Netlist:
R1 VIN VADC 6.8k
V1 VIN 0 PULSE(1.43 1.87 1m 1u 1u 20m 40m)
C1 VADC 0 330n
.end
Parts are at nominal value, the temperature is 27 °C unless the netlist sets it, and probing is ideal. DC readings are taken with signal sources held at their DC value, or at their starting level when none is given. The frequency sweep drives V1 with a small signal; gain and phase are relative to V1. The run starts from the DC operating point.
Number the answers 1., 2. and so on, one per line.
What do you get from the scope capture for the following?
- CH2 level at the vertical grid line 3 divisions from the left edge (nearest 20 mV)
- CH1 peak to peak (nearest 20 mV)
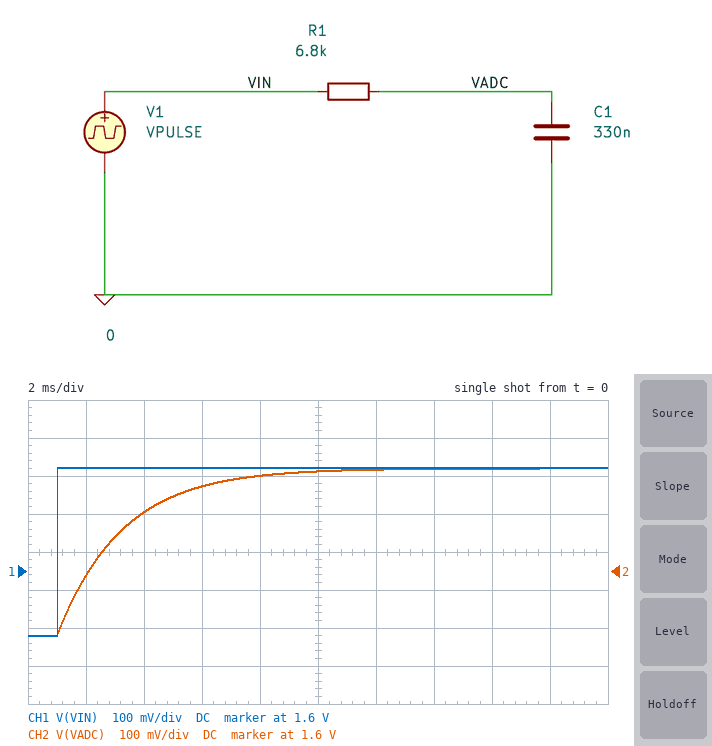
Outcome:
1. 1.82 V
2. 440 mV
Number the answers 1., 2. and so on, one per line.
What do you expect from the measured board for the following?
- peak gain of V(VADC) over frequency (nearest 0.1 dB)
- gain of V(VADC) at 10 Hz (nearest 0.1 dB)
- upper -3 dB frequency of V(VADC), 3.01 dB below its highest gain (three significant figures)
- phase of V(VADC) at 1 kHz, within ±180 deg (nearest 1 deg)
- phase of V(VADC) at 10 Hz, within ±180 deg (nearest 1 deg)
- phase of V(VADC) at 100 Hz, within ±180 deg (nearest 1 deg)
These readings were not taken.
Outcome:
1. 0 dB
2. -0.1 dB
3. 70.9 Hz
4. -86 deg
5. -8 deg
6. -55 deg
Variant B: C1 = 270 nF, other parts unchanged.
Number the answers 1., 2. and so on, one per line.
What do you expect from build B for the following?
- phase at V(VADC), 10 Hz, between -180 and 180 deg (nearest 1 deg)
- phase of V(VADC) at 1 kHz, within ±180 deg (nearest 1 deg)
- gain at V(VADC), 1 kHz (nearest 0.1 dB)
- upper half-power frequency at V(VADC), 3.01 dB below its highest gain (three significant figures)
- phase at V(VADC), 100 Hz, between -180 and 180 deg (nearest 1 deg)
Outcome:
1. -7 deg
2. -85 deg
3. -21.3 dB
4. 86.7 Hz
5. -49 deg
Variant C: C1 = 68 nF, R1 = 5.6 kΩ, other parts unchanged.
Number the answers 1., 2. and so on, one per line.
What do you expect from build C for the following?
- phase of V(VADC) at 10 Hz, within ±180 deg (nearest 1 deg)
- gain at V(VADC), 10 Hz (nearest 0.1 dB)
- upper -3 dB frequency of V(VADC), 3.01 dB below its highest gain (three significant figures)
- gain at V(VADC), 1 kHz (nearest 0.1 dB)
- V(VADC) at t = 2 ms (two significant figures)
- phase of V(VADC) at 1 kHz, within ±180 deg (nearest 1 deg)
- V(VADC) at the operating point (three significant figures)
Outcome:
1. -1 deg
2. 0 dB
3. 418 Hz
4. -8.3 dB
5. 1.8 V
6. -67 deg
7. 1.43 V
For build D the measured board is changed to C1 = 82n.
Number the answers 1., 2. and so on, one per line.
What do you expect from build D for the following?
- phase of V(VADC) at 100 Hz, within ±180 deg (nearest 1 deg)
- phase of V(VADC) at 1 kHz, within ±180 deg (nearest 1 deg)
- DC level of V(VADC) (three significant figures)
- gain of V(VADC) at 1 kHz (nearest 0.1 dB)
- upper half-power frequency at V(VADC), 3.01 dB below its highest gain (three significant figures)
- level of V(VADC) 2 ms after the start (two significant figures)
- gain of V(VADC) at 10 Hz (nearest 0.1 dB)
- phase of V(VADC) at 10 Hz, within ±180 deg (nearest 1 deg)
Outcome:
1. -19 deg
2. -74 deg
3. 1.43 V
4. -11.2 dB
5. 285 Hz
6. 1.8 V
7. 0 dB
8. -2 deg
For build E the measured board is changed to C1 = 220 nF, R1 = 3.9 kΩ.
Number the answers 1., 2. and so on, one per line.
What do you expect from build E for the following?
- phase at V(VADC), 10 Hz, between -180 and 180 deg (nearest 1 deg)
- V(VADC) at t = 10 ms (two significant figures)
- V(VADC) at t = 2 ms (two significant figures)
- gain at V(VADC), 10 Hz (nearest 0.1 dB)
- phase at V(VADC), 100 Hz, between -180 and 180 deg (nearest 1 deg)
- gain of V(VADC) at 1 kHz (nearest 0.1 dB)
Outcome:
1. -3 deg
2. 1.9 V
3. 1.7 V
4. 0 dB
5. -28 deg
6. -14.8 dB
